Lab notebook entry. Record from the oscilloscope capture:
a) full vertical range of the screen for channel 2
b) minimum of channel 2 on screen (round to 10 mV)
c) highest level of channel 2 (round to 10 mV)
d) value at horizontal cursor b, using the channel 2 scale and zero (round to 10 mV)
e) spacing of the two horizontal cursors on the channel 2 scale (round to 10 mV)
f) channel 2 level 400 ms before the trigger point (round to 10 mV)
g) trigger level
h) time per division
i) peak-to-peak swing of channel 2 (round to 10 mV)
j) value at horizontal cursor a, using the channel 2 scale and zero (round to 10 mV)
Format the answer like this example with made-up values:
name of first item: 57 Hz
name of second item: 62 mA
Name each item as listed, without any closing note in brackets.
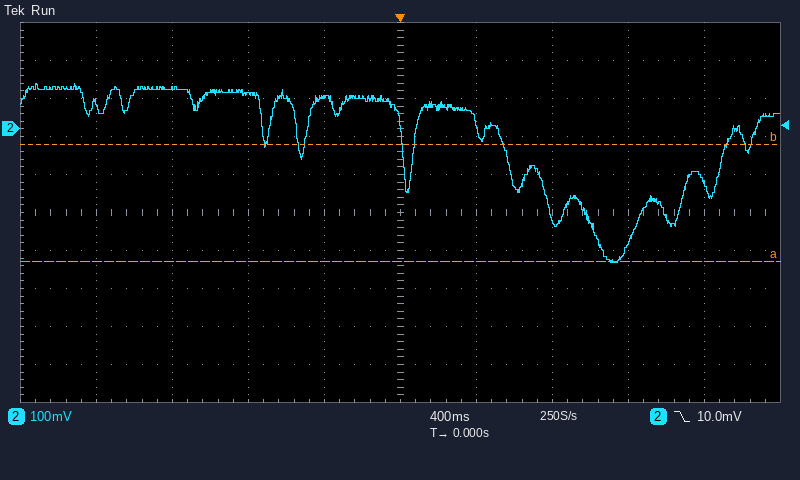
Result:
full vertical range of the screen for channel 2: 1 V
minimum of channel 2 on screen: -350 mV
highest level of channel 2: 120 mV
value at horizontal cursor b, using the channel 2 scale and zero: -40 mV
spacing of the two horizontal cursors on the channel 2 scale: 310 mV
channel 2 level 400 ms before the trigger point: 80 mV
trigger level: 10.0 mV
time per division: 400 ms
peak-to-peak swing of channel 2: 470 mV
value at horizontal cursor a, using the channel 2 scale and zero: -350 mV
